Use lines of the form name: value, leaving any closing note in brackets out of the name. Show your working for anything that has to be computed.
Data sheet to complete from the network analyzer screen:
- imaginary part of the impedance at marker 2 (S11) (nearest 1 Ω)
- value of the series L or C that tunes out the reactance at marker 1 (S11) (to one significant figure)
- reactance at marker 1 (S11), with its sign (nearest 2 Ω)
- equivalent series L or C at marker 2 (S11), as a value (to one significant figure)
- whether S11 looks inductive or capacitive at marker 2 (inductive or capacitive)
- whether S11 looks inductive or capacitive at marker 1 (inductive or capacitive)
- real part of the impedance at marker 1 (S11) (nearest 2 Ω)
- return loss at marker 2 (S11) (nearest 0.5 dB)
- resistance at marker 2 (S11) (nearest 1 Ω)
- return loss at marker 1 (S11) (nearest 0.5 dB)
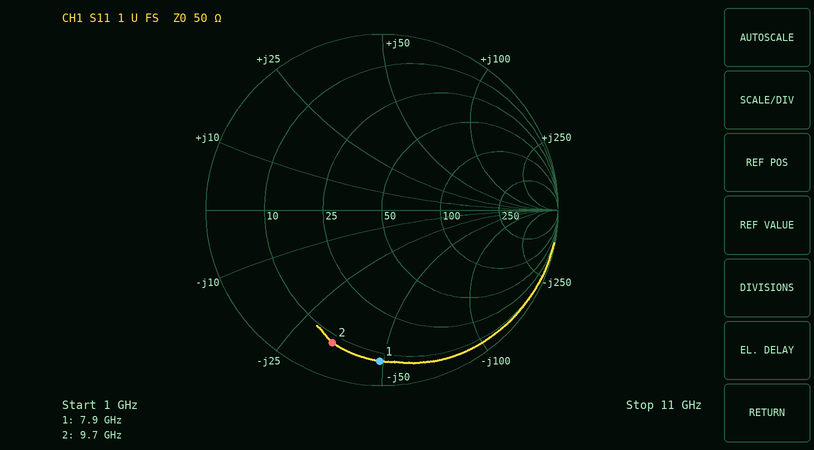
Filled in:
imaginary part of the impedance at marker 2 (S11): -34 Ω
value of the series L or C that tunes out the reactance at marker 1 (S11): L = 48 Ω/(2π × 7.9 GHz) ≈ 1.0 nH
reactance at marker 1 (S11), with its sign: -48 Ω
equivalent series L or C at marker 2 (S11), as a value: C = 1/(2π × 9.7 GHz × 34 Ω) ≈ 483 fF, so 500 fF to one significant figure
whether S11 looks inductive or capacitive at marker 2: capacitive
whether S11 looks inductive or capacitive at marker 1: capacitive
real part of the impedance at marker 1 (S11): 8 Ω
return loss at marker 2 (S11): 2.0 dB
resistance at marker 2 (S11): 8 Ω
return loss at marker 1 (S11): 1.5 dB
